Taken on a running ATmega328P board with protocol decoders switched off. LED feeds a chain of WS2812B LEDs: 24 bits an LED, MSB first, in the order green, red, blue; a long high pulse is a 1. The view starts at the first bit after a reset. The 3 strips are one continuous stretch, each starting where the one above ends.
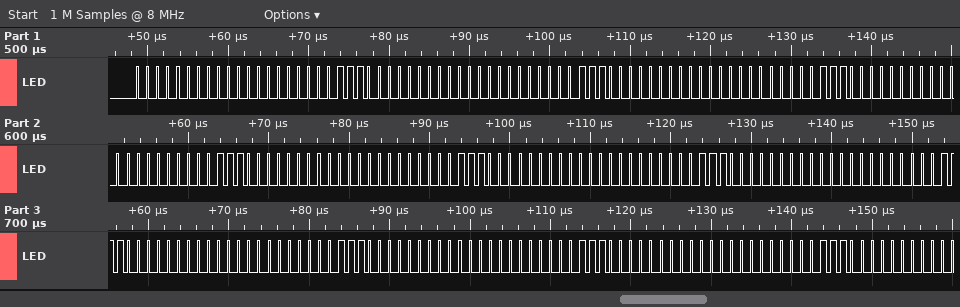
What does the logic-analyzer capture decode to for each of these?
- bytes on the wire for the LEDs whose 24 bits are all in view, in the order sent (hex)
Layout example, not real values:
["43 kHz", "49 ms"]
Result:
["00 00 0E 00 00 0E 00 00 0E 00 00 0E 00 00 0E 00 00 0E 00 00 0E 00 00 0E 00 00 0E 00 00 0E"]
